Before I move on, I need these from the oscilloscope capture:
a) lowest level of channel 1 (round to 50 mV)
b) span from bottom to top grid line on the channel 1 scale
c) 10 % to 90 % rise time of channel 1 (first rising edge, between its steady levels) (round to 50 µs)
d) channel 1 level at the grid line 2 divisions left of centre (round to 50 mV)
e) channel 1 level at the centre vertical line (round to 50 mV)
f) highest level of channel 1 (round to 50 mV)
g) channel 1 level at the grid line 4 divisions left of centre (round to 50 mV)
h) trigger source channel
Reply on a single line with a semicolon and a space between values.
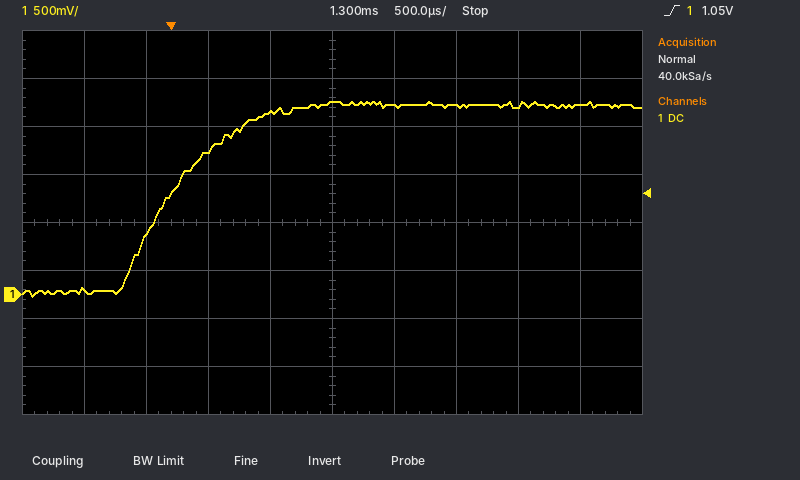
0 mV; 4 V; 950 µs; 1.50 V; 2.00 V; 2.00 V; 50 mV; channel 1
